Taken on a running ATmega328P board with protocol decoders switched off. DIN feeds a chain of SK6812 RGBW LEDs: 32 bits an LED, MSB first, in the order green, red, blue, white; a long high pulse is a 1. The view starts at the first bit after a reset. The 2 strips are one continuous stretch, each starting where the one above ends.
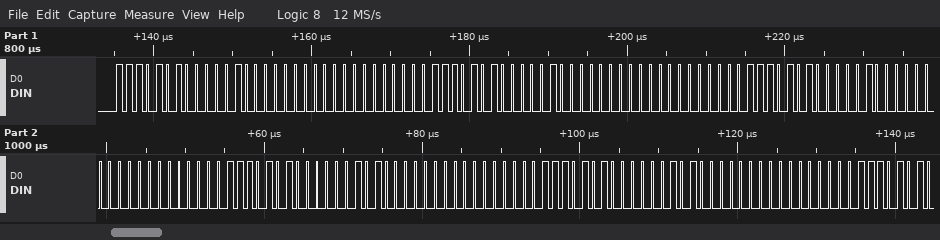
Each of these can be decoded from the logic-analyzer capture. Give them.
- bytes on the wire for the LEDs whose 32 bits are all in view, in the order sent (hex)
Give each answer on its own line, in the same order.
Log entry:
EA 08 00 00 EA 08 00 00 EA 08 00 00 EA 05 00 00 EA 05 00 00
